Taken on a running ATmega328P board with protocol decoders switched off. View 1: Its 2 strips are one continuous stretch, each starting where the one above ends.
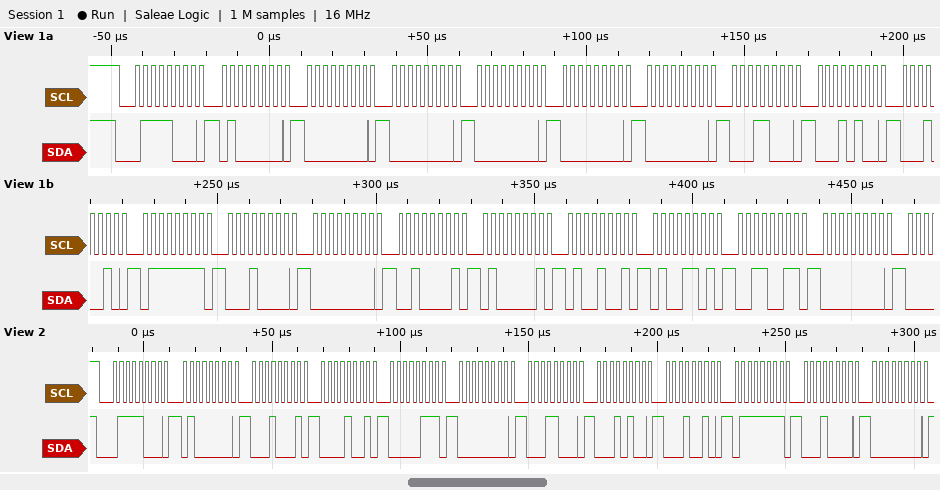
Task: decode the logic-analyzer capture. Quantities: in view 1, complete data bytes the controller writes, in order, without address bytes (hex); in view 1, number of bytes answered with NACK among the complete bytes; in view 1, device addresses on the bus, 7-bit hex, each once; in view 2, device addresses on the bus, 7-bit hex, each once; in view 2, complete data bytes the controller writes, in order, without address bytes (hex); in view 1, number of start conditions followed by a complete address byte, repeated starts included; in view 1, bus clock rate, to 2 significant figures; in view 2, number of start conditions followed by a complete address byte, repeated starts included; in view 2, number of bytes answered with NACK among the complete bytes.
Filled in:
40 00 00 00 00 00 18 14 12 7F 10 00 21 41 49 4D 33 00
0
0x3C
0x3C
40 11 09 07 00 18 14 12 7F 10 00
1
400 kHz
1
0
